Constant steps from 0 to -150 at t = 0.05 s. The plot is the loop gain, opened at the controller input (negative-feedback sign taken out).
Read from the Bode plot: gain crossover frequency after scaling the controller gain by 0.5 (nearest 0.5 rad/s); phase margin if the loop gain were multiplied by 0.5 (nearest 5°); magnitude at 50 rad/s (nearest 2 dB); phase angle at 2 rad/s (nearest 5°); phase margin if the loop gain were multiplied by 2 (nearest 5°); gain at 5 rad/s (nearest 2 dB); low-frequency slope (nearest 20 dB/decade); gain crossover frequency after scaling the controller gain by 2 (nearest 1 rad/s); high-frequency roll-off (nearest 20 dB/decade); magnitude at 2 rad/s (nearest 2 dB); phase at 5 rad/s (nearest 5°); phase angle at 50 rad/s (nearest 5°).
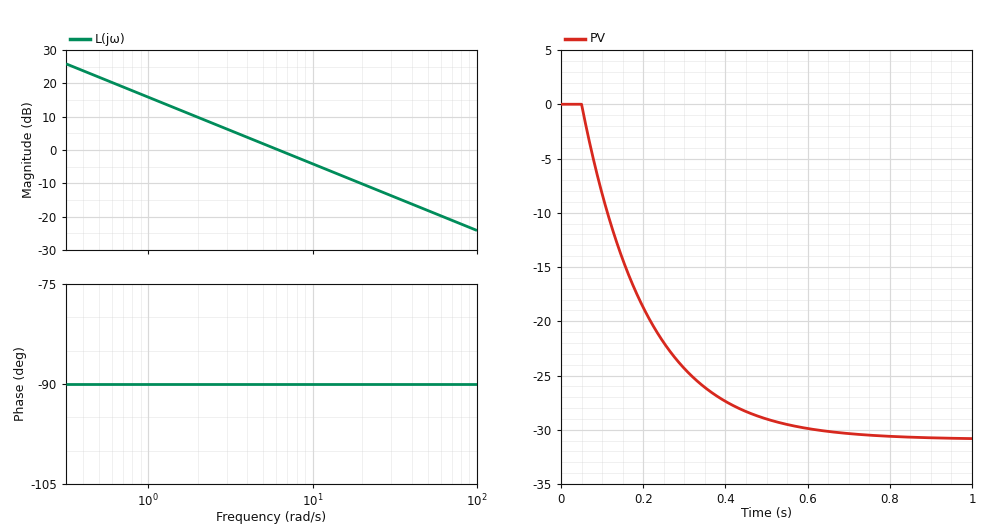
3.0 rad/s
90°
-18 dB
-90°
90°
2 dB
-20 dB/decade
12 rad/s
-20 dB/decade
10 dB
-90°
-90°
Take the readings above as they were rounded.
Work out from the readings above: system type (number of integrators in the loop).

1
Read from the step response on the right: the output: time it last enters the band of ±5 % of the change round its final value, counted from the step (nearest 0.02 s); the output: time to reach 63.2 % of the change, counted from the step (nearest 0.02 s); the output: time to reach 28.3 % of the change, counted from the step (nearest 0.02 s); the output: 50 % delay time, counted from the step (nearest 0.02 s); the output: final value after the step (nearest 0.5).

0.48 s
0.16 s
0.06 s
0.12 s
-31.0
